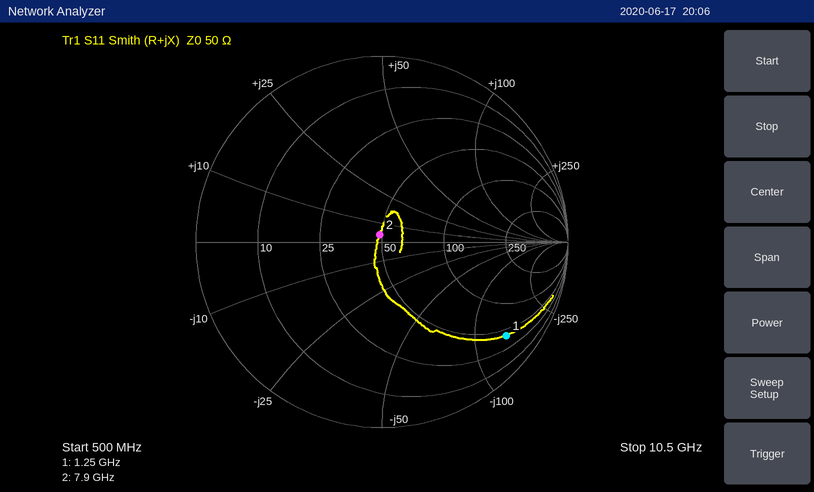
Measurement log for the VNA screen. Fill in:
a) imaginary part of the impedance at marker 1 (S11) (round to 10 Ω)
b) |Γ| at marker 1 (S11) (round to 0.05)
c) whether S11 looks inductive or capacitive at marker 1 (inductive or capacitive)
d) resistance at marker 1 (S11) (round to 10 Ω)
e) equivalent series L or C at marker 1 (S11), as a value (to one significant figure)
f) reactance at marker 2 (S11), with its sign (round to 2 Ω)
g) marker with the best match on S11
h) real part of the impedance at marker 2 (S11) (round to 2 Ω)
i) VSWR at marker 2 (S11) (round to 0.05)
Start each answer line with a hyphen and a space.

- -140 Ω
- 0.85
- capacitive
- 40 Ω
- 900 fF
- +4 Ω
- marker 2
- 48 Ω
- 1.10
